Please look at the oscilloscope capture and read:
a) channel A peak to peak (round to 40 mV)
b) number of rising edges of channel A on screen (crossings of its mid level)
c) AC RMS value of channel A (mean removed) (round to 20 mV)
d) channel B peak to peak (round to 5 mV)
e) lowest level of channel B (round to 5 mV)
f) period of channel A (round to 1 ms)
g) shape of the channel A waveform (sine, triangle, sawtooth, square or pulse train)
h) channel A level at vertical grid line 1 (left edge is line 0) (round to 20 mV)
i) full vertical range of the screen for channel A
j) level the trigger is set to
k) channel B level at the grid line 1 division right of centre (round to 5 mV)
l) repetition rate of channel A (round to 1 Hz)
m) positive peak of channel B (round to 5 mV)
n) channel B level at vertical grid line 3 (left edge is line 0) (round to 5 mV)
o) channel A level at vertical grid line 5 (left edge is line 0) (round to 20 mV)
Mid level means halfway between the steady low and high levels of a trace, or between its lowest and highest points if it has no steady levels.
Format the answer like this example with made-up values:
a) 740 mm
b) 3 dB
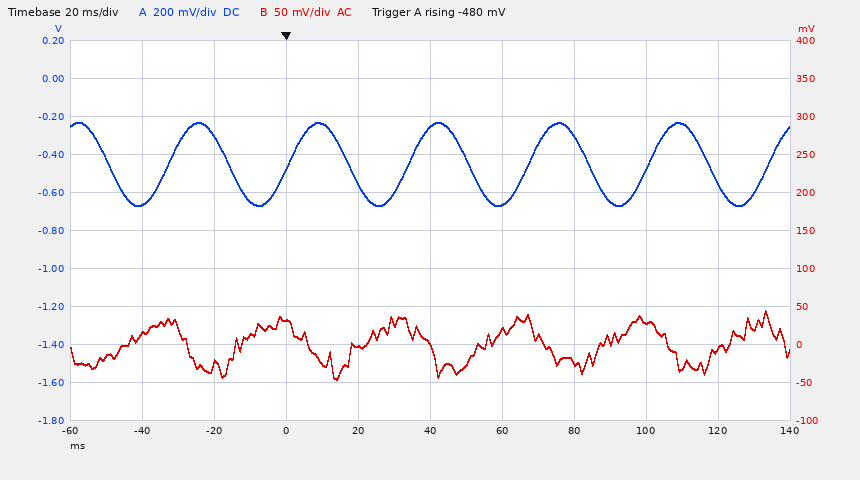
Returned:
a) 440 mV
b) 6
c) 160 mV
d) 90 mV
e) -45 mV
f) 33 ms
g) sine
h) -660 mV
i) 2 V
j) -480 mV
k) 20 mV
l) 30 Hz
m) 45 mV
n) 30 mV
o) -260 mV
